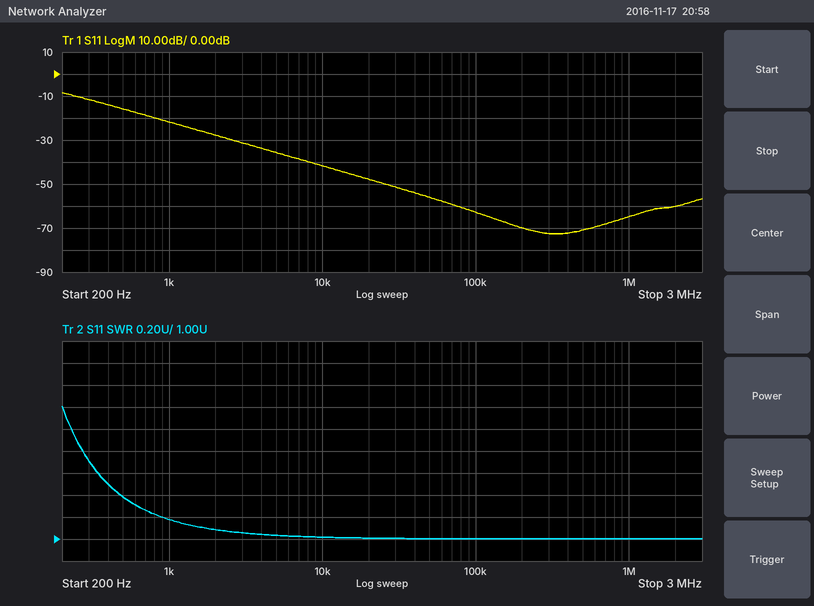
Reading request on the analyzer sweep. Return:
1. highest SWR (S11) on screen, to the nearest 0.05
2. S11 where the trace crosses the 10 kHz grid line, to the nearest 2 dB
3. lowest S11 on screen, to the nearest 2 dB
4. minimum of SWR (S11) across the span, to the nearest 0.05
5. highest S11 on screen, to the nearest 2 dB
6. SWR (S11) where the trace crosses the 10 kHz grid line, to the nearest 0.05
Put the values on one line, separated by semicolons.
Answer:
2.20; -42 dB; -72 dB; 1.00; -8 dB; 1.00
